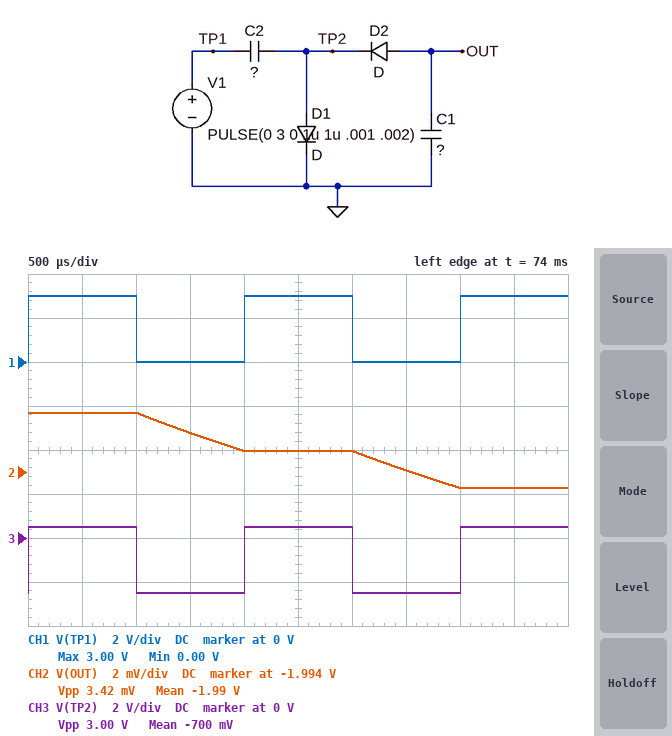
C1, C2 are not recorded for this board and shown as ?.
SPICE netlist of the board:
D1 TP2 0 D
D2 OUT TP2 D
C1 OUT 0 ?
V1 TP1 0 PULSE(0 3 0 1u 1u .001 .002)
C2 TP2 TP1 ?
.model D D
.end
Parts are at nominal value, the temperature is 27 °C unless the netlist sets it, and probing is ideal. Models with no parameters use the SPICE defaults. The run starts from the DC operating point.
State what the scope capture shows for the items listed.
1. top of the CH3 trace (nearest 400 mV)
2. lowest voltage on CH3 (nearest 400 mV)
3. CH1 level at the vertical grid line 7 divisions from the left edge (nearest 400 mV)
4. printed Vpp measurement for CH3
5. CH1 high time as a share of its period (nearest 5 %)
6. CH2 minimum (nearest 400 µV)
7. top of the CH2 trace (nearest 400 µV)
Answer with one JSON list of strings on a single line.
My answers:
["400 mV", "-2.4 V", "0 V", "3.00 V", "50 %", "-1.9948 V", "-1.9912 V"]
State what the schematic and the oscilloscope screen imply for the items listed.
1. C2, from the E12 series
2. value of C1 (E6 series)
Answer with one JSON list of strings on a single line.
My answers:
["680 nF", "1.5 µF"]
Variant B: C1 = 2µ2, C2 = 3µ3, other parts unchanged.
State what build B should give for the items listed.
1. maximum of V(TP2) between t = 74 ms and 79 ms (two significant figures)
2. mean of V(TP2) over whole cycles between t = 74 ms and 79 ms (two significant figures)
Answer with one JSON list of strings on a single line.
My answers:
["520 mV", "-980 mV"]
